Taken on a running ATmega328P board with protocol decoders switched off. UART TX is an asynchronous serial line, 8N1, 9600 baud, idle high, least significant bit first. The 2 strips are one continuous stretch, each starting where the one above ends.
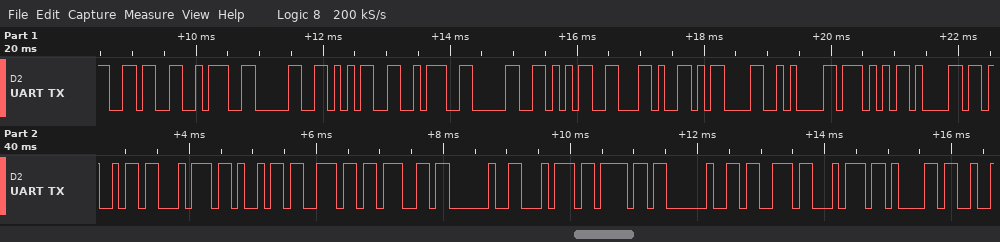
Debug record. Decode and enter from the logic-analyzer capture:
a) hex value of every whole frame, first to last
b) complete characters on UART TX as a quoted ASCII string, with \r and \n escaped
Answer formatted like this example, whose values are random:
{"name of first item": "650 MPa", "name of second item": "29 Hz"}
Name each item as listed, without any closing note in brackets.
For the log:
{"hex value of every whole frame, first to last": "36 3A 30 35 3A 30 35 2C 0D 0A 57 61 69 74 69 6E 67 20 74 6F 20 73 74 61", "complete characters on UART TX as a quoted ASCII string, with \\r and \\n escaped": "\"6:05:05,\\r\\nWaiting to sta\""}
